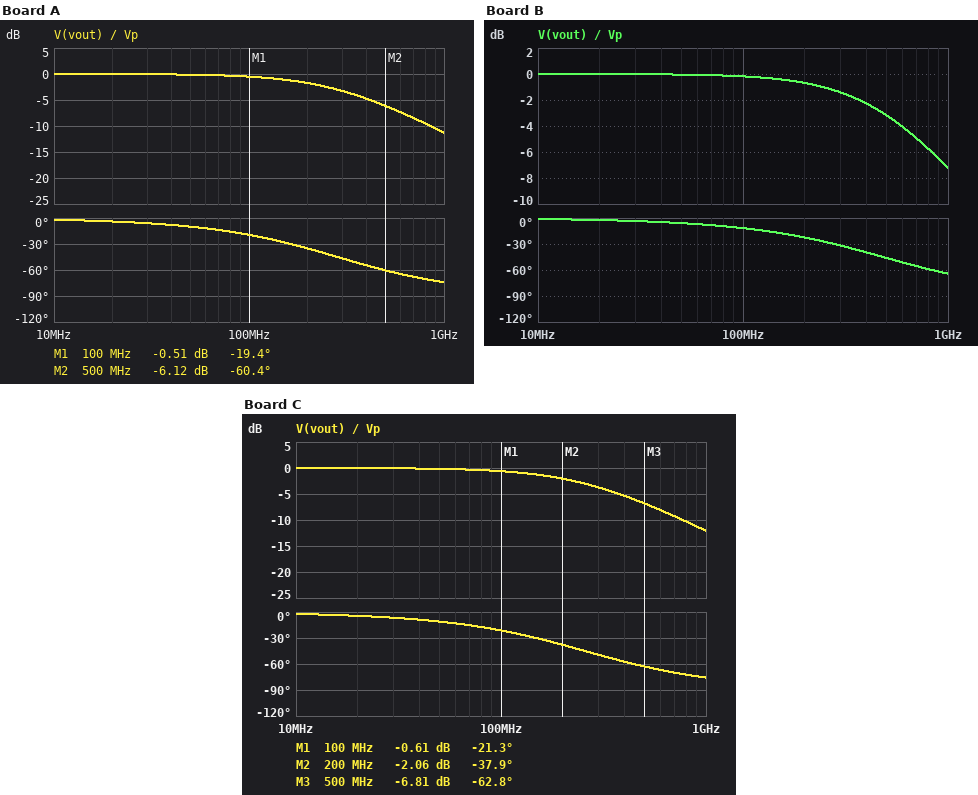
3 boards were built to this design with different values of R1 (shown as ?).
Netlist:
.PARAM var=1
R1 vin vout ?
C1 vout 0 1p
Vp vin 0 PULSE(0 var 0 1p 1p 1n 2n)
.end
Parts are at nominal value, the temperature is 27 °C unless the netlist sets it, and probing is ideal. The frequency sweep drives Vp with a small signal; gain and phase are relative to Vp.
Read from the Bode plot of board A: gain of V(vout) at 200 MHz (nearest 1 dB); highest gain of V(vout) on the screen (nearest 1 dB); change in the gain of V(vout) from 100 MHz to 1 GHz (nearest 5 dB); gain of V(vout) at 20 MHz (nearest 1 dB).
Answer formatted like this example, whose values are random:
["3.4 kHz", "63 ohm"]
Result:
["-2 dB", "0 dB", "-10 dB", "0 dB"]
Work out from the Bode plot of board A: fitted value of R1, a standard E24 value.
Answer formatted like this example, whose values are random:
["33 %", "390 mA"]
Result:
["560 Ω"]
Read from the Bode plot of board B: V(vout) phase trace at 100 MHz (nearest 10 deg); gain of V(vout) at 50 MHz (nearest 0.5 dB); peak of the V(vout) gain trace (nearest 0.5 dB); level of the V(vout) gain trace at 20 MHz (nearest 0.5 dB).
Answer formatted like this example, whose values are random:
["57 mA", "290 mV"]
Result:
["-10 deg", "0 dB", "0 dB", "0 dB"]
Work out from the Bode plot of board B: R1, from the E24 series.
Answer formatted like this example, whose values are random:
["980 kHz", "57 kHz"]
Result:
["330 Ω"]
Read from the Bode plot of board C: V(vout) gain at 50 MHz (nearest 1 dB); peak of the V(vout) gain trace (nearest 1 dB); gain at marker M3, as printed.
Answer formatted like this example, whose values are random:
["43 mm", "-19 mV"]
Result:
["0 dB", "0 dB", "-6.81 dB"]
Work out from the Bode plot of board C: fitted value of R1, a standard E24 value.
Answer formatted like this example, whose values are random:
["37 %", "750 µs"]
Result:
["620 Ω"]
